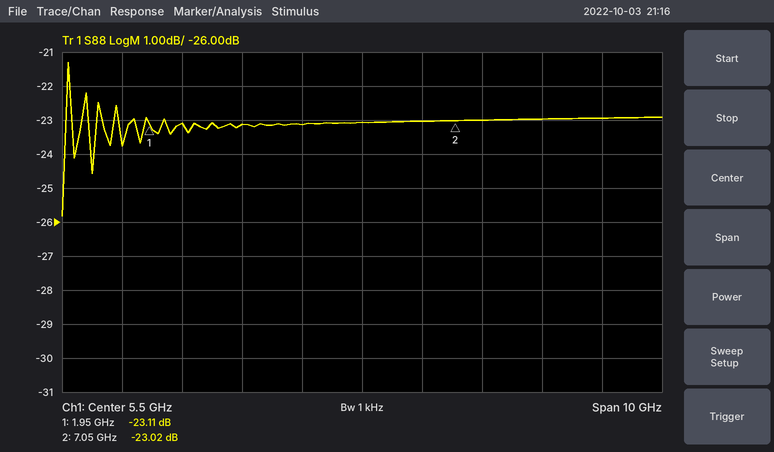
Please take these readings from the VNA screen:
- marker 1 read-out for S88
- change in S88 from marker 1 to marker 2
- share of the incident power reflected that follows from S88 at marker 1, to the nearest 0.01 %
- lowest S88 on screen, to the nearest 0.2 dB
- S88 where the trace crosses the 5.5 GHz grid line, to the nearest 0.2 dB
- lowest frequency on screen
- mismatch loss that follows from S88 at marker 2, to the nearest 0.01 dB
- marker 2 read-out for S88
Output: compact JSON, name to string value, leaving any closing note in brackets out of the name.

{"marker 1 read-out for S88": "-23.11 dB", "change in S88 from marker 1 to marker 2": "0.09 dB", "share of the incident power reflected that follows from S88 at marker 1, to the nearest 0.01 %": "0.49 %", "lowest S88 on screen, to the nearest 0.2 dB": "-25.8 dB", "S88 where the trace crosses the 5.5 GHz grid line, to the nearest 0.2 dB": "-23.0 dB", "lowest frequency on screen": "500 MHz", "mismatch loss that follows from S88 at marker 2, to the nearest 0.01 dB": "0.02 dB", "marker 2 read-out for S88": "-23.02 dB"}
